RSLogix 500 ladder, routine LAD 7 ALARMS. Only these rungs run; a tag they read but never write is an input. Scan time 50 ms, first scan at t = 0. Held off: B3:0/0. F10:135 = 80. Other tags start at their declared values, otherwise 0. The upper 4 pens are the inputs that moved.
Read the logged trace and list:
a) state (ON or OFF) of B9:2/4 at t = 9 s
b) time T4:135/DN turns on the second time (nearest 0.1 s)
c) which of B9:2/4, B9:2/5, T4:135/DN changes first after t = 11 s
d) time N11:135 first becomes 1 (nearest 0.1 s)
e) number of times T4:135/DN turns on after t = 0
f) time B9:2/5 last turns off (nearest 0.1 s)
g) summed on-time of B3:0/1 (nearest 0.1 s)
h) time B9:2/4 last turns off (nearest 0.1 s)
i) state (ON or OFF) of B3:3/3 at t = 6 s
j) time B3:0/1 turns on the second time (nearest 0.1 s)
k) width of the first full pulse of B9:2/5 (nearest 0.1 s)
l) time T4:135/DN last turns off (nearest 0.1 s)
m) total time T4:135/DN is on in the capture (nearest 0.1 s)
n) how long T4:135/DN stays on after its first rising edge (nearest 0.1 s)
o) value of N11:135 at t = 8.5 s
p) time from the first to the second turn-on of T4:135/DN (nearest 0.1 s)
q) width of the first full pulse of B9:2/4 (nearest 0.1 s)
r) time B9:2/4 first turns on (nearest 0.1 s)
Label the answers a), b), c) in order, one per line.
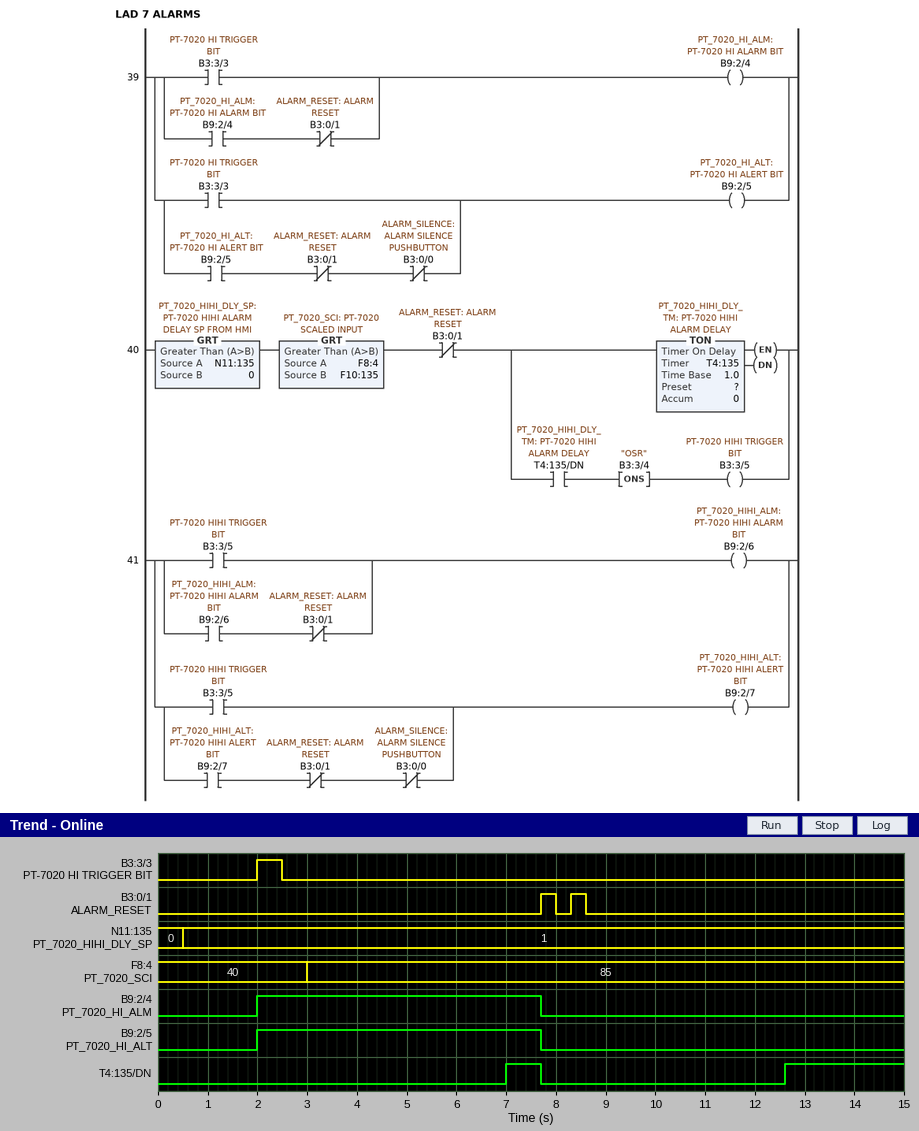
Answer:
a) OFF
b) 12.6 s
c) T4:135/DN
d) 0.5 s
e) 2
f) 7.7 s
g) 0.6 s
h) 7.7 s
i) OFF
j) 8.3 s
k) 5.7 s
l) 7.7 s
m) 3.1 s
n) 0.7 s
o) 1
p) 5.6 s
q) 5.7 s
r) 2.0 s
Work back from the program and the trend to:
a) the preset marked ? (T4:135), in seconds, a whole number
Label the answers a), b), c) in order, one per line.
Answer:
a) 4 s
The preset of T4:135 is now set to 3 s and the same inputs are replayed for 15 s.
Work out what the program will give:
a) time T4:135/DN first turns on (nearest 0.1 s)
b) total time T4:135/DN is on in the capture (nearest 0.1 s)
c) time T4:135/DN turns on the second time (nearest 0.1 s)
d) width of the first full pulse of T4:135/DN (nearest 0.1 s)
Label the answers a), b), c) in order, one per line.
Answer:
a) 6.0 s
b) 5.1 s
c) 11.6 s
d) 1.7 s
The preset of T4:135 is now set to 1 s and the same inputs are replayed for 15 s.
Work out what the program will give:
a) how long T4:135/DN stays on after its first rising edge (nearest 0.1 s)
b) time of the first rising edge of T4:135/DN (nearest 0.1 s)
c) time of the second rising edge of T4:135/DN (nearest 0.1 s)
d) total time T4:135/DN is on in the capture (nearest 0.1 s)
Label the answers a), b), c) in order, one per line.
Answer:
a) 3.7 s
b) 4.0 s
c) 9.6 s
d) 9.1 s
